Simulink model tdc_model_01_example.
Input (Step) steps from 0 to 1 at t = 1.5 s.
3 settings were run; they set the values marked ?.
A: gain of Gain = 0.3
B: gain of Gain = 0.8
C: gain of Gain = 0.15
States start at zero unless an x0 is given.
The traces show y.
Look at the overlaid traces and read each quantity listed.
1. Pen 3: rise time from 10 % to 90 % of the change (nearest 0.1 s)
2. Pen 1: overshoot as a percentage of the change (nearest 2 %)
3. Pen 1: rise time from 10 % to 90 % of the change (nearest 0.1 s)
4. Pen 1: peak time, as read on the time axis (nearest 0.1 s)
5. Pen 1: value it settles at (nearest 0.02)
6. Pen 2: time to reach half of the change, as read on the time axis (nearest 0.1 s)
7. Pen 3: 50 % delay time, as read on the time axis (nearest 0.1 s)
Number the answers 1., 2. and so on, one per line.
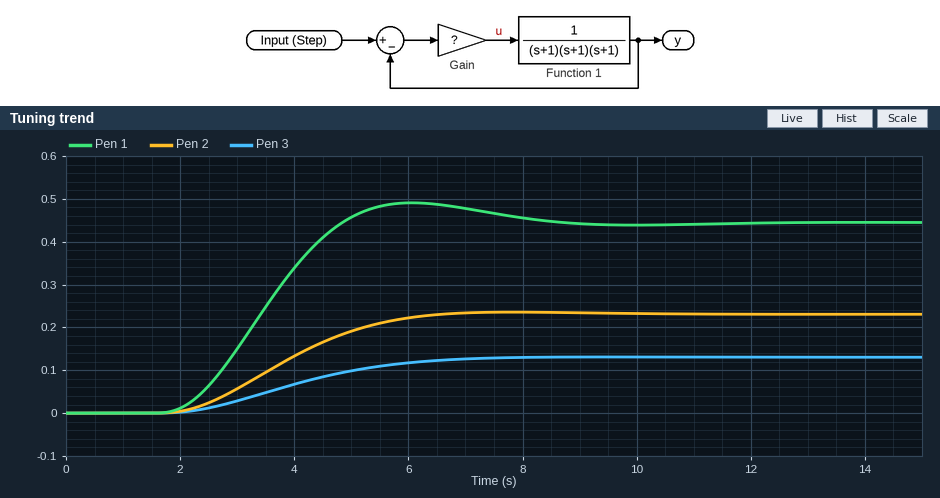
1. 3.5 s
2. 10 %
3. 2.1 s
4. 6.1 s
5. 0.44
6. 3.8 s
7. 3.9 s
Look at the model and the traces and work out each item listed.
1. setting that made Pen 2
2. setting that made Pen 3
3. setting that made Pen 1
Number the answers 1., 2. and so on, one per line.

1. A
2. C
3. B
